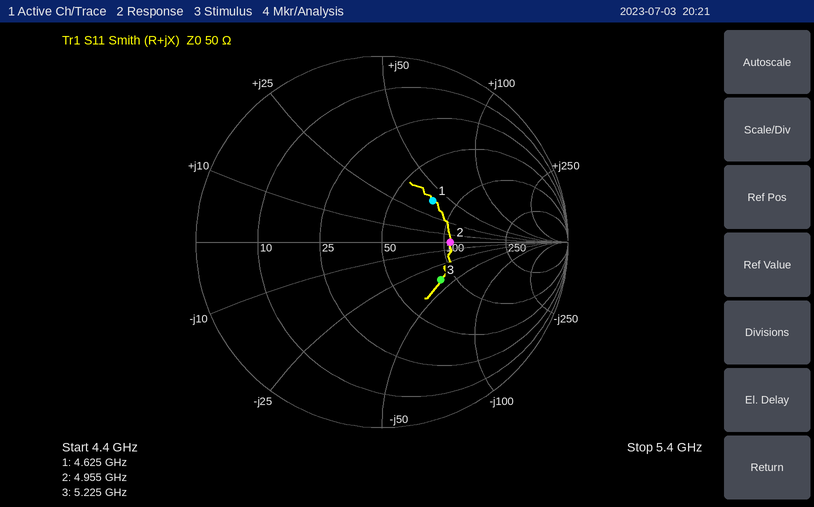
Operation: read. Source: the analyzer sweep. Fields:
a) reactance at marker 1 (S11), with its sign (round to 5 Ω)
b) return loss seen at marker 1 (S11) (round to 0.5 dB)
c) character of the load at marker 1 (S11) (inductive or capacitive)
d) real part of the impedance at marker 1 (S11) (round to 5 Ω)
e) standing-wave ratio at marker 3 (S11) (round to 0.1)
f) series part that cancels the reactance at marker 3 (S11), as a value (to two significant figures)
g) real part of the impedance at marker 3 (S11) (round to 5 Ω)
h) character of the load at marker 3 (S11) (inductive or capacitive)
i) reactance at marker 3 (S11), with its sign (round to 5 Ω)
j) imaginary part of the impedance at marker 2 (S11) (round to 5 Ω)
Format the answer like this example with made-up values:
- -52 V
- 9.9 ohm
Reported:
- +40 Ω
- 9.0 dB
- inductive
- 75 Ω
- 2.2
- 1.2 nH
- 85 Ω
- capacitive
- -40 Ω
- 0 Ω
